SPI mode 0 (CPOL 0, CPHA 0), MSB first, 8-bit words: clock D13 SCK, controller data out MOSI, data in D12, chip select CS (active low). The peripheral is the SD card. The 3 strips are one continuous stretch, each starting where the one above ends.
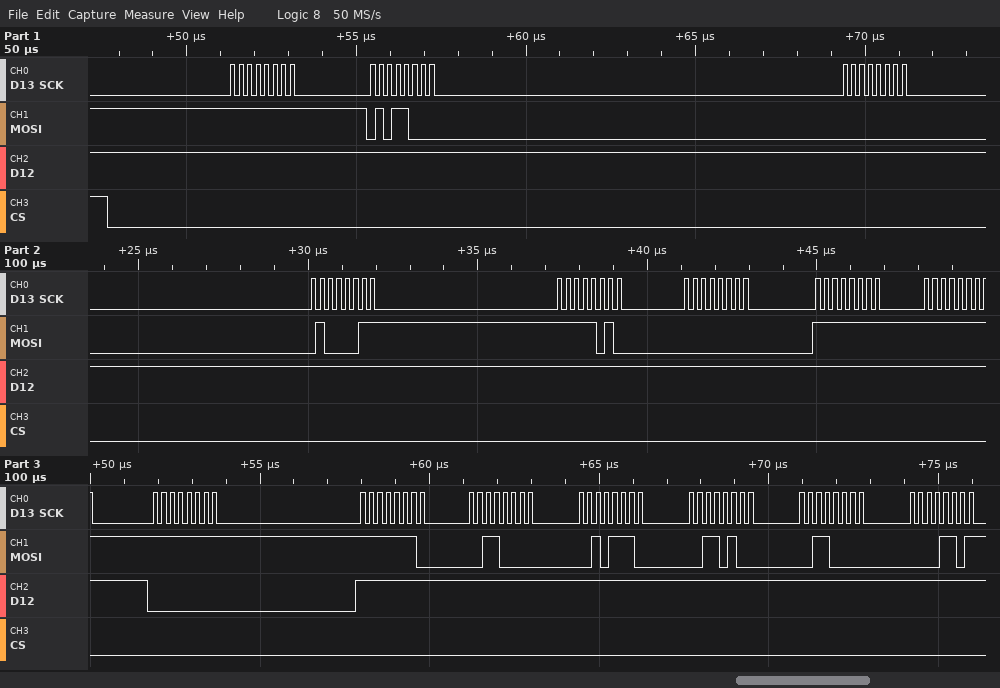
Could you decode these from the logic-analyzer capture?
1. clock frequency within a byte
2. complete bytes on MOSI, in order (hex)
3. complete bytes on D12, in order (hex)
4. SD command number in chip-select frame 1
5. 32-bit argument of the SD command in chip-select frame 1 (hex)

4 MHz
FF 58 00 43 FA 00 FF FF FF FE 30 2E 34 30 0D
FF FF FF FF FF FF FF FF 00 FF FF FF FF FF FF
CMD24
0x0043FA00
